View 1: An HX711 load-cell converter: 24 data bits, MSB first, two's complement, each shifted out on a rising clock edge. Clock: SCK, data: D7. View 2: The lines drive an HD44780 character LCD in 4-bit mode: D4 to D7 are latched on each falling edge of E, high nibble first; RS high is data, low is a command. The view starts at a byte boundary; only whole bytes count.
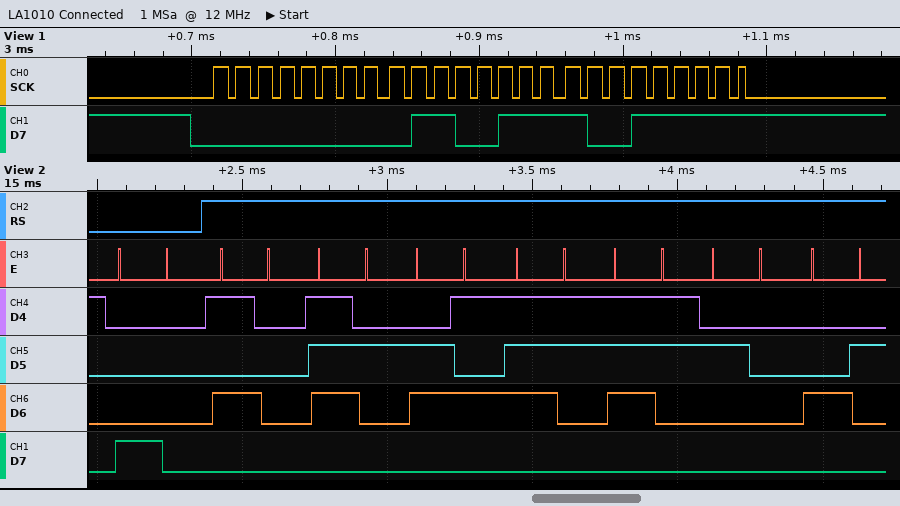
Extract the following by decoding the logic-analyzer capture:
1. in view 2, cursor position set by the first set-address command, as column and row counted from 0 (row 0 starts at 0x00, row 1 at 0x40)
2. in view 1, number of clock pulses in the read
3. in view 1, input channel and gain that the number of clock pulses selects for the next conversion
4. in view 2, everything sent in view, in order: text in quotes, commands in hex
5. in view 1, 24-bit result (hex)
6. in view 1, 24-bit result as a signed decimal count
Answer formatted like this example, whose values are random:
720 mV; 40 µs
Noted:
column 0, row 0; 25; channel A, gain 128; 0x80 "Press B"; 0x00679F; 26527
